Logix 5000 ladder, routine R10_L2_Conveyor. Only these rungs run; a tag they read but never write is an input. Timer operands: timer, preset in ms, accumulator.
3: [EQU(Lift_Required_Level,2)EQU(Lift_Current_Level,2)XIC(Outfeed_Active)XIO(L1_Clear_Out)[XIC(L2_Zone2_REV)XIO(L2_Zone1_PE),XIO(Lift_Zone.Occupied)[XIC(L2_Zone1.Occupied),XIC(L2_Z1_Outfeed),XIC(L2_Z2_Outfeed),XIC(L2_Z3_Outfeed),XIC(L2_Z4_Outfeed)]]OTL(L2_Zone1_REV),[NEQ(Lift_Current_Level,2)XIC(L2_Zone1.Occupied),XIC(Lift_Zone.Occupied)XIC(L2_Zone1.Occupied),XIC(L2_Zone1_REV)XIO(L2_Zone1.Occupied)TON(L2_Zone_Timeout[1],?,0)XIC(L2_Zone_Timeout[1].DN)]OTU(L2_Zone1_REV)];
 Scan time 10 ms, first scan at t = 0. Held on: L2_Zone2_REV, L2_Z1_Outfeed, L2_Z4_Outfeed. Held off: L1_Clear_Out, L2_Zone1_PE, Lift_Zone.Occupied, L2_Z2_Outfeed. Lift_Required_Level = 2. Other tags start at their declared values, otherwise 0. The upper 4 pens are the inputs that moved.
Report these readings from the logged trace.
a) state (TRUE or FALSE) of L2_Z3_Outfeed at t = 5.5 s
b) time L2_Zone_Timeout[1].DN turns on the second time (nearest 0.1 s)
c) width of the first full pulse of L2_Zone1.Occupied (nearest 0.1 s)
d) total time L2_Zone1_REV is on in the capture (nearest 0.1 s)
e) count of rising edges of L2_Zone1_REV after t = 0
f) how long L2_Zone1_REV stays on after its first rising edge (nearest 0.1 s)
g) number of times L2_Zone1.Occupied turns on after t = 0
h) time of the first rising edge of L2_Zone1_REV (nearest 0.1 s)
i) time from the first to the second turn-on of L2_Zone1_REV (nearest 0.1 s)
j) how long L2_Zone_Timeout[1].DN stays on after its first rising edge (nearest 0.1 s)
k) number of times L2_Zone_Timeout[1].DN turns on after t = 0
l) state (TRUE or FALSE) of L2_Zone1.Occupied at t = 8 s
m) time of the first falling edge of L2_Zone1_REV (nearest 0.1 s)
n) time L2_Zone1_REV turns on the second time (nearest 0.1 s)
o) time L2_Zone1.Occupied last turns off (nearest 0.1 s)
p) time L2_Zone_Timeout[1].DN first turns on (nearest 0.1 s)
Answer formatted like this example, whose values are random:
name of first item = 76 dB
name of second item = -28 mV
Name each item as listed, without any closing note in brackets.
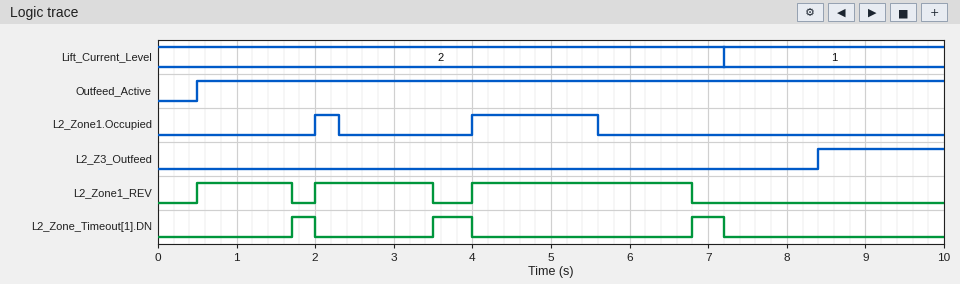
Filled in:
state (TRUE or FALSE) of L2_Z3_Outfeed at t = 5.5 s = FALSE
time L2_Zone_Timeout[1].DN turns on the second time = 3.5 s
width of the first full pulse of L2_Zone1.Occupied = 0.3 s
total time L2_Zone1_REV is on in the capture = 5.5 s
count of rising edges of L2_Zone1_REV after t = 0 = 3
how long L2_Zone1_REV stays on after its first rising edge = 1.2 s
number of times L2_Zone1.Occupied turns on after t = 0 = 2
time of the first rising edge of L2_Zone1_REV = 0.5 s
time from the first to the second turn-on of L2_Zone1_REV = 1.5 s
how long L2_Zone_Timeout[1].DN stays on after its first rising edge = 0.3 s
number of times L2_Zone_Timeout[1].DN turns on after t = 0 = 3
state (TRUE or FALSE) of L2_Zone1.Occupied at t = 8 s = FALSE
time of the first falling edge of L2_Zone1_REV = 1.7 s
time L2_Zone1_REV turns on the second time = 2.0 s
time L2_Zone1.Occupied last turns off = 5.6 s
time L2_Zone_Timeout[1].DN first turns on = 1.7 s
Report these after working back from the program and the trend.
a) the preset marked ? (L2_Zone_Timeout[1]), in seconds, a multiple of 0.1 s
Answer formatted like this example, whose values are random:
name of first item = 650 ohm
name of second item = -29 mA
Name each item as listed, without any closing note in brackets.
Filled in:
the preset marked ? (L2_Zone_Timeout[1]), in seconds, a multiple of 0.1 s = 1.2 s
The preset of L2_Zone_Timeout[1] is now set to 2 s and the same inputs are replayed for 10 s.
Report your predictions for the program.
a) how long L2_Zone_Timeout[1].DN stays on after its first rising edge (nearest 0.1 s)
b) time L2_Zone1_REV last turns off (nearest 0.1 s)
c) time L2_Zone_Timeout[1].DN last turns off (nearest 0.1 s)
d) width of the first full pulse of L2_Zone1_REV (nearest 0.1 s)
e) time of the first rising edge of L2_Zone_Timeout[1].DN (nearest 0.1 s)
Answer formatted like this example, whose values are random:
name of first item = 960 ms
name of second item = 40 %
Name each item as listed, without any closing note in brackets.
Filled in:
how long L2_Zone_Timeout[1].DN stays on after its first rising edge = 0.0 s
time L2_Zone1_REV last turns off = 7.6 s
time L2_Zone_Timeout[1].DN last turns off = 7.6 s
width of the first full pulse of L2_Zone1_REV = 7.1 s
time of the first rising edge of L2_Zone_Timeout[1].DN = 7.6 s
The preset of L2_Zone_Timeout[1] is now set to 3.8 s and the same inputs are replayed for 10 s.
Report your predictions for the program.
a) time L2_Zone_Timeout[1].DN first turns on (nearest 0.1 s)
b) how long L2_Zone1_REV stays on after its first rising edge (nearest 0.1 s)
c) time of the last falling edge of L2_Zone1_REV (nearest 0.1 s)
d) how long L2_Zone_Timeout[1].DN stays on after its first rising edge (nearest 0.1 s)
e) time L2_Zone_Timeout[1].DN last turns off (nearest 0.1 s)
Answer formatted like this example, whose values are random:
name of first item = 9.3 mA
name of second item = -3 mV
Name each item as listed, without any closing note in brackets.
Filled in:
time L2_Zone_Timeout[1].DN first turns on = 9.4 s
how long L2_Zone1_REV stays on after its first rising edge = 8.9 s
time of the last falling edge of L2_Zone1_REV = 9.4 s
how long L2_Zone_Timeout[1].DN stays on after its first rising edge = 0.0 s
time L2_Zone_Timeout[1].DN last turns off = 9.4 s
